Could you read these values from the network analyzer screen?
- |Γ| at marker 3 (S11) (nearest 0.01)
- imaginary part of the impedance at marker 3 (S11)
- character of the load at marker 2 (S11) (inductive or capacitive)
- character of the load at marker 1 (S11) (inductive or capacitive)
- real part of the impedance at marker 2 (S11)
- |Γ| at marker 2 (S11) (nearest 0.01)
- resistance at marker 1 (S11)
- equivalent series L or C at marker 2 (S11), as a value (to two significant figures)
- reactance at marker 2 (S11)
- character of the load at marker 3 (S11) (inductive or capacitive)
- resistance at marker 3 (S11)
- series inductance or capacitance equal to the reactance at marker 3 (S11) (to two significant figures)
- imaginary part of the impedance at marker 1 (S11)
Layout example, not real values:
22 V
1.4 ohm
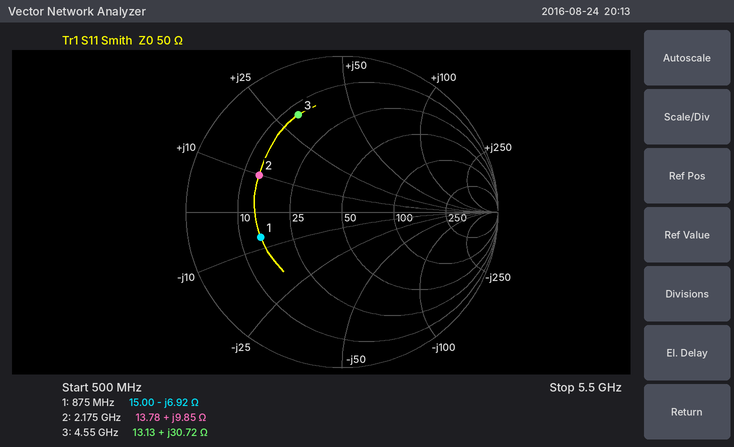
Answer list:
0.68
+30.72 Ω
inductive
capacitive
13.78 Ω
0.58
15.00 Ω
720 pH
+9.85 Ω
inductive
13.13 Ω
1.1 nH
-6.92 Ω
